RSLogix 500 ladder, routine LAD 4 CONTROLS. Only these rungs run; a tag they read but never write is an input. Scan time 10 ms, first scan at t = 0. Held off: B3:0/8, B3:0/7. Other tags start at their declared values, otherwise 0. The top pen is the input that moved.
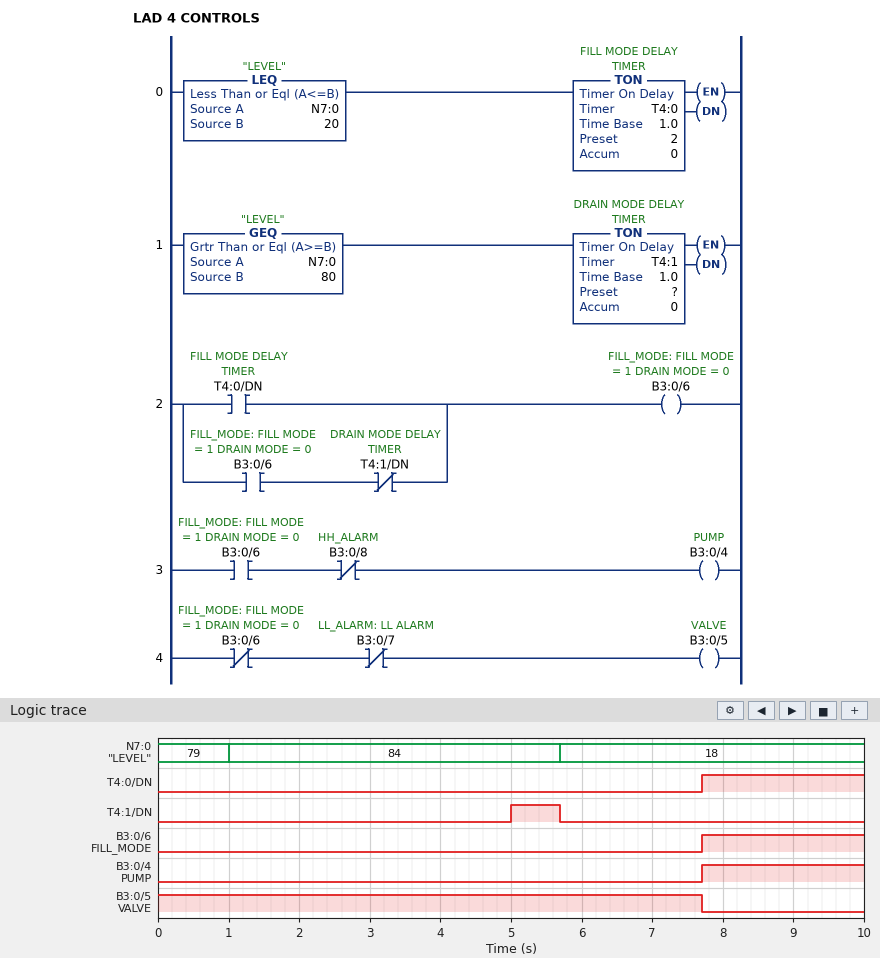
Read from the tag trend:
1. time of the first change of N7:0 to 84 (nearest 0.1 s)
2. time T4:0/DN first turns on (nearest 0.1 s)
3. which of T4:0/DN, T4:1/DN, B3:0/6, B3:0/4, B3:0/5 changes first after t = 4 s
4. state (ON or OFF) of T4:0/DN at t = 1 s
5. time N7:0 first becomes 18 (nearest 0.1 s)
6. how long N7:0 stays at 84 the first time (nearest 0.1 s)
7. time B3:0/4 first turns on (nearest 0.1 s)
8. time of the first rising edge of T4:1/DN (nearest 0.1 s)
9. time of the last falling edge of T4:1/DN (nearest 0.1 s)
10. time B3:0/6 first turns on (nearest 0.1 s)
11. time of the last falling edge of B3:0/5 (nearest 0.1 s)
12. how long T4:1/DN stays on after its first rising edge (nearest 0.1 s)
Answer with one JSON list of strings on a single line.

["1.0 s", "7.7 s", "T4:1/DN", "OFF", "5.7 s", "4.7 s", "7.7 s", "5.0 s", "5.7 s", "7.7 s", "7.7 s", "0.7 s"]
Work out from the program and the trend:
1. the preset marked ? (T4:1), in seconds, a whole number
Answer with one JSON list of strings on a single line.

["4 s"]
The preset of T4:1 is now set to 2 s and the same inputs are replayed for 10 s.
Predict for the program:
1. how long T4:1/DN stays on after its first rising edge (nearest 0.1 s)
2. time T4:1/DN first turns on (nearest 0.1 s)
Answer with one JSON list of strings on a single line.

["2.7 s", "3.0 s"]
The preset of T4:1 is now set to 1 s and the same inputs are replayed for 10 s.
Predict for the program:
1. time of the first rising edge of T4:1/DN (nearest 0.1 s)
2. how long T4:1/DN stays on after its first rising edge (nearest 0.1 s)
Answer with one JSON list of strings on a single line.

["2.0 s", "3.7 s"]
